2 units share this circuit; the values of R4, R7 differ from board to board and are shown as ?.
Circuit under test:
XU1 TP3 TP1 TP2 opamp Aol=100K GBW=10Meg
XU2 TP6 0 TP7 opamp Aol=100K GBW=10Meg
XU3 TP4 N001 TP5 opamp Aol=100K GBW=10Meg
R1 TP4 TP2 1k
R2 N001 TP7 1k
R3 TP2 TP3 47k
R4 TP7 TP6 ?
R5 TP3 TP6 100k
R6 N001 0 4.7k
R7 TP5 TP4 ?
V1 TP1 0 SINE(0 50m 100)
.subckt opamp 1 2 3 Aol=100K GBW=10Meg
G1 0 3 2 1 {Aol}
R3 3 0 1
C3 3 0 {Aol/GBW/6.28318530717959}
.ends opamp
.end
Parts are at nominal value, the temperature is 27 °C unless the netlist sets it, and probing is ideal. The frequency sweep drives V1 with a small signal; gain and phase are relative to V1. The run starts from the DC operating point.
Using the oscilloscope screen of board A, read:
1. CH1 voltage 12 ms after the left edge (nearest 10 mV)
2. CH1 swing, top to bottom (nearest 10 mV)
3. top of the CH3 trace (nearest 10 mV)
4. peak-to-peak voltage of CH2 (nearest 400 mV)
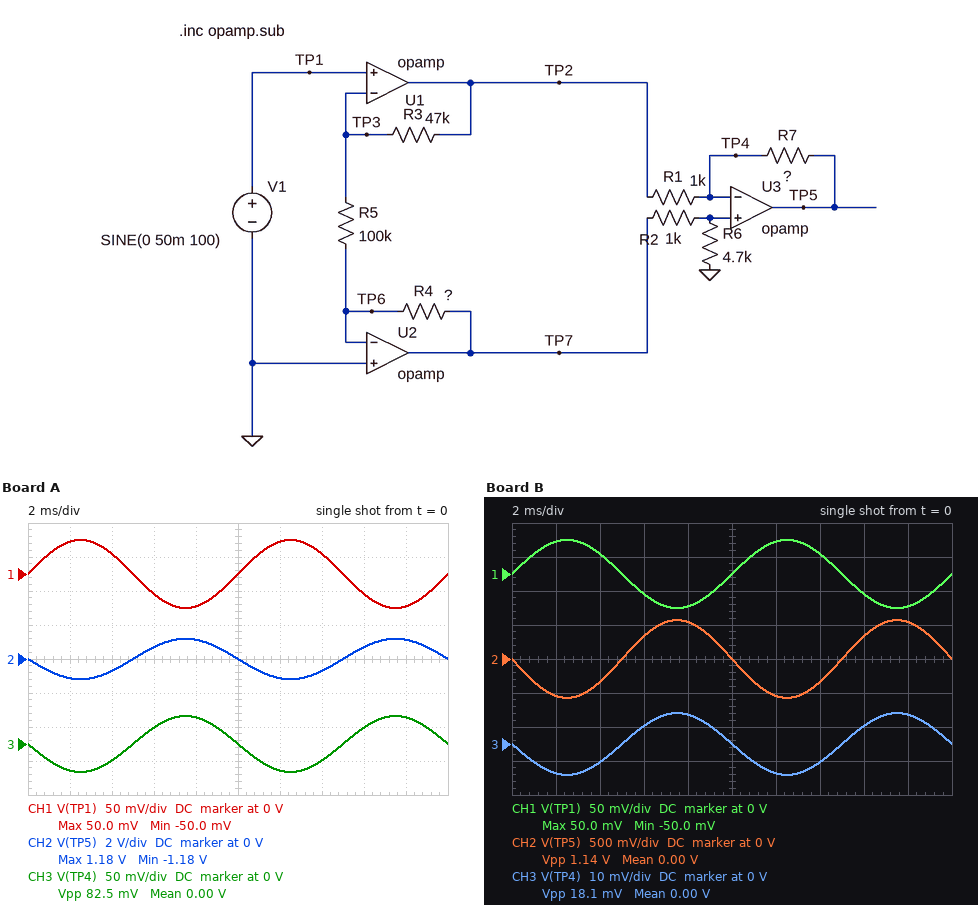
50 mV
100 mV
40 mV
2.4 V
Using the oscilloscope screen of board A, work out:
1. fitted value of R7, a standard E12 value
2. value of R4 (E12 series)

10 kΩ
100 kΩ
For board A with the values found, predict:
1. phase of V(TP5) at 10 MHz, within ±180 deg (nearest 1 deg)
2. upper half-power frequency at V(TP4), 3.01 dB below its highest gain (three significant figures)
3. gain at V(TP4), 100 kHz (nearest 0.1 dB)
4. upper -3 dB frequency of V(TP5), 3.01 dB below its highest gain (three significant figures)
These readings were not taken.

28 deg
6.74 MHz
-1.6 dB
869 kHz
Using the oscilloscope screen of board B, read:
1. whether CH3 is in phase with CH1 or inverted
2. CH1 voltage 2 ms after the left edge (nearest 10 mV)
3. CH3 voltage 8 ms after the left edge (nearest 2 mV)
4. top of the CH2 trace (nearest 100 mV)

inverted
50 mV
8 mV
600 mV
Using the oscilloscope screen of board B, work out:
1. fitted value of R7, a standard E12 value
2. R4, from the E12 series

6.8 kΩ
22 kΩ
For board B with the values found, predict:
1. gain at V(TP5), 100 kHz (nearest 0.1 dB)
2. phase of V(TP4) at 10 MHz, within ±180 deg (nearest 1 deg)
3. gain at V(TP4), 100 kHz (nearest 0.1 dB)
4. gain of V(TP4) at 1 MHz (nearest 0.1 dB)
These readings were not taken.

21.1 dB
-48 deg
-13.7 dB
-1.9 dB
